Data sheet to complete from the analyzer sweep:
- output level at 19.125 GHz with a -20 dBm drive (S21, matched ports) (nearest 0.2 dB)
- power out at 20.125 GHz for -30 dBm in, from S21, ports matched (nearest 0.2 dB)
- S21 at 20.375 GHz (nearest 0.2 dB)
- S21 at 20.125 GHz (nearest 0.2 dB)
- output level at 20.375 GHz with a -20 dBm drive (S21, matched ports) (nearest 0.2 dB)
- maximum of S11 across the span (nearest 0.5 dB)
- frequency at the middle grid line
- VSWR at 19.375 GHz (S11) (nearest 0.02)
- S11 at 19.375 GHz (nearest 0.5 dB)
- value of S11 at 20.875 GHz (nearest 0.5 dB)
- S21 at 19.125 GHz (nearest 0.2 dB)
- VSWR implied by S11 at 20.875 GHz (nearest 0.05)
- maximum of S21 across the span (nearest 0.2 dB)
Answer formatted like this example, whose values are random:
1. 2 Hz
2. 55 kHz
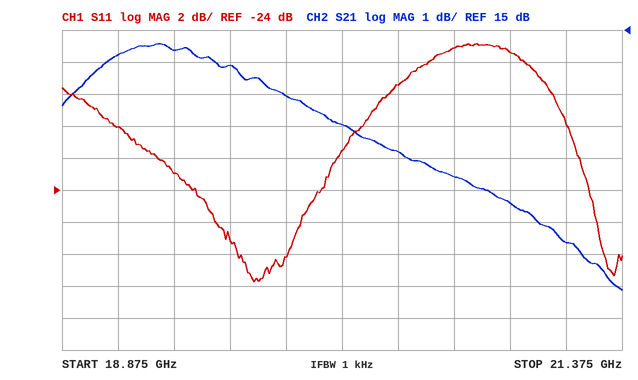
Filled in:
1. -5.8 dBm
2. -18.0 dBm
3. 11.2 dB
4. 12.0 dB
5. -8.8 dBm
6. -15.0 dB
7. 20.125 GHz
8. 1.16
9. -23.0 dB
10. -15.5 dB
11. 14.2 dB
12. 1.40
13. 14.6 dB
